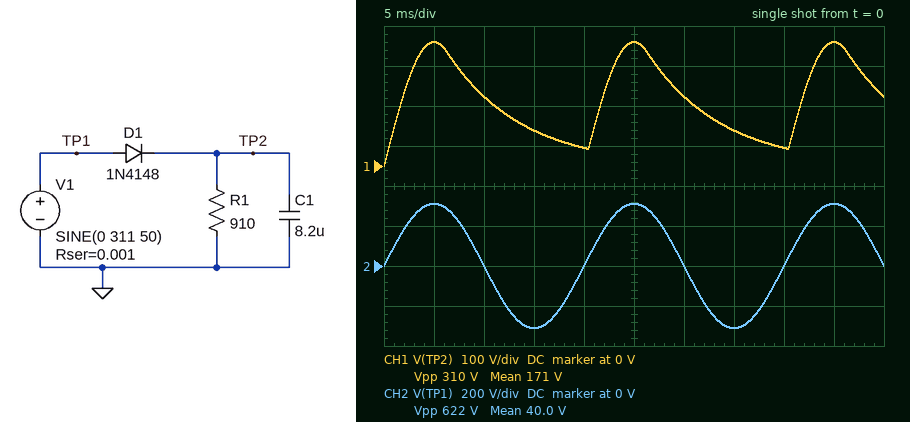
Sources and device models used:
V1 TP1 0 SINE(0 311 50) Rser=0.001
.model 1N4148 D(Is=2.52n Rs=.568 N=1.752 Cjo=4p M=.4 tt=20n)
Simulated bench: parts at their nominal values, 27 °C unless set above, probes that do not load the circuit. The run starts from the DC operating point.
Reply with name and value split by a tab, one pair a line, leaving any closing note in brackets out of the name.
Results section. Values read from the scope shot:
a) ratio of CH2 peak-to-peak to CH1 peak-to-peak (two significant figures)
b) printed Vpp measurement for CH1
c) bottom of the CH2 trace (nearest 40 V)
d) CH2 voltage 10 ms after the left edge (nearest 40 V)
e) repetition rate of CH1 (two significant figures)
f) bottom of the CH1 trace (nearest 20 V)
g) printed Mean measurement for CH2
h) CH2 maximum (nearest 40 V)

ratio of CH2 peak-to-peak to CH1 peak-to-peak	2.0
printed Vpp measurement for CH1	310 V
bottom of the CH2 trace	-320 V
CH2 voltage 10 ms after the left edge	0 V
repetition rate of CH1	50 Hz
bottom of the CH1 trace	0 V
printed Mean measurement for CH2	40.0 V
CH2 maximum	320 V
